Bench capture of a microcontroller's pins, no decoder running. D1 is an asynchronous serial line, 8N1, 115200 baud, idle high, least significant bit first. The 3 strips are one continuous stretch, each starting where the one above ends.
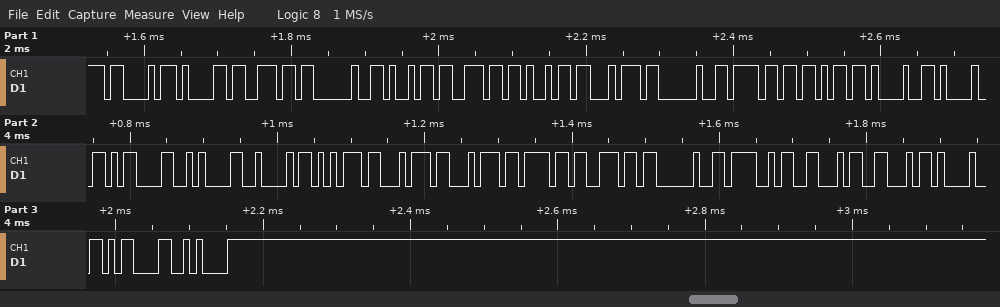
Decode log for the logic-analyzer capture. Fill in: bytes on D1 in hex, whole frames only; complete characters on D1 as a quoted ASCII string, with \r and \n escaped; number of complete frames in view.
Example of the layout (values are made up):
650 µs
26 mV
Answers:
43 61 6E 20 69 6E 69 74 20 6F 6B 21 21 0D 0A 42 75 74 74 6F 6E 20 4F 46 46 21 0D 0A
"Can init ok!!\r\nButton OFF!\r\n"
28
